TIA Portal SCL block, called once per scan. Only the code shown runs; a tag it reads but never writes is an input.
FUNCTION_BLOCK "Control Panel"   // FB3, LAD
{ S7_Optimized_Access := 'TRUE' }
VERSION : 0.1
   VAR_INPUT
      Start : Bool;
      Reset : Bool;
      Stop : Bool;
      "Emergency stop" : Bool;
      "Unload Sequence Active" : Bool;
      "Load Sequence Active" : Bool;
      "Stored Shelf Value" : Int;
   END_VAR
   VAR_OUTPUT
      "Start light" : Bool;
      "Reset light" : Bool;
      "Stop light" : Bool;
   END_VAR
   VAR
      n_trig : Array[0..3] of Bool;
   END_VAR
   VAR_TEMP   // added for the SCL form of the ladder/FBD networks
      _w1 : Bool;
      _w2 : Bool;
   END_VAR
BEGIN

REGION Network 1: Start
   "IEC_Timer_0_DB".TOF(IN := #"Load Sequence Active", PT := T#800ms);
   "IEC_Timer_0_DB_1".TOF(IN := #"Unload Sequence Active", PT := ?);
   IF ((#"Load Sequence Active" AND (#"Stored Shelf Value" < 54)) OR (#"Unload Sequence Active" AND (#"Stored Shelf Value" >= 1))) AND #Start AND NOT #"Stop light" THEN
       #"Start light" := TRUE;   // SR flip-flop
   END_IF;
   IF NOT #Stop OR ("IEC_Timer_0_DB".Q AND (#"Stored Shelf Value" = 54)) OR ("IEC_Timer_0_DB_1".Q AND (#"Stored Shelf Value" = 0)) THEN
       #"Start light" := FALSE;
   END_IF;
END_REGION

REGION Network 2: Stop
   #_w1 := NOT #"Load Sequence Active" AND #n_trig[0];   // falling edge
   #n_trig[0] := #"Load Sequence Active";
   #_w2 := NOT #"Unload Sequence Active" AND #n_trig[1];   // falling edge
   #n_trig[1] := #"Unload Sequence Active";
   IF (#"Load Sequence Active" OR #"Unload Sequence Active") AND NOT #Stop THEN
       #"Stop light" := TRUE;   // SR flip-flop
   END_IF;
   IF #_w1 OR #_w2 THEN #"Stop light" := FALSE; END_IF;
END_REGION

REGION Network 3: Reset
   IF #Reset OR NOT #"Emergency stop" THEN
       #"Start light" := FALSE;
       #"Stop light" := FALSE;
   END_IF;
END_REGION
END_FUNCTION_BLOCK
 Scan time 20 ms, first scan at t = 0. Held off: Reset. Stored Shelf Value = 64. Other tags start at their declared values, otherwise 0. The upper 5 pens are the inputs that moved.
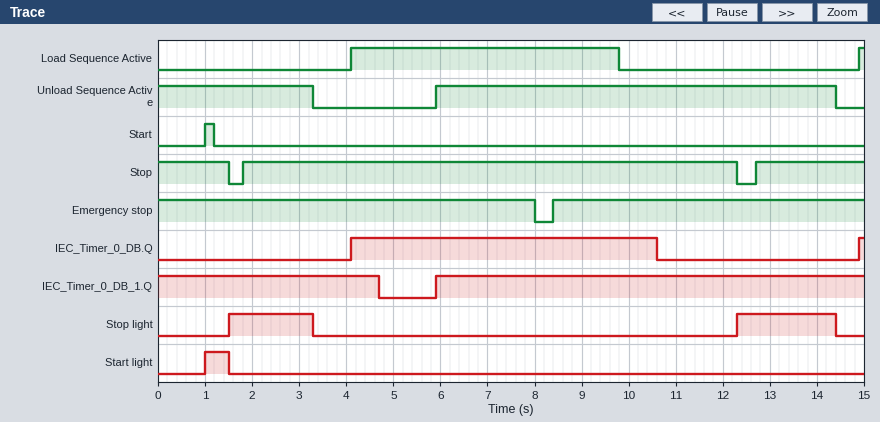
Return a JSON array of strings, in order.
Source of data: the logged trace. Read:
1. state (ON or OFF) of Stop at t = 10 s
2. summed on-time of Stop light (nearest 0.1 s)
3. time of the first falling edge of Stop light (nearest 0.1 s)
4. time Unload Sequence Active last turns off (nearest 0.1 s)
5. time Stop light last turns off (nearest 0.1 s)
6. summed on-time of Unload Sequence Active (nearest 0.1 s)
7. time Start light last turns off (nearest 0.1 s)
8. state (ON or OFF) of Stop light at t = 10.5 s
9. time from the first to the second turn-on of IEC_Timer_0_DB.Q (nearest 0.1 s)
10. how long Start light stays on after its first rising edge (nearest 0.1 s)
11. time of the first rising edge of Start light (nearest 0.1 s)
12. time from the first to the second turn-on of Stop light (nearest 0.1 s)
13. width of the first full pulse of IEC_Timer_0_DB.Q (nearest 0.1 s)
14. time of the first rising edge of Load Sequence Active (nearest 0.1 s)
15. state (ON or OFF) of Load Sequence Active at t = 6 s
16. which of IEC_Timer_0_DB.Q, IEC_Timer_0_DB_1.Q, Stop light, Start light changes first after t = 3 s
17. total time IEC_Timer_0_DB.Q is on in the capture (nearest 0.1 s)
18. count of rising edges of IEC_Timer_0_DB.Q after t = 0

["ON", "3.9 s", "3.3 s", "14.4 s", "14.4 s", "11.8 s", "1.5 s", "OFF", "10.8 s", "0.5 s", "1.0 s", "10.8 s", "6.5 s", "4.1 s", "ON", "Stop light", "6.6 s", "2"]
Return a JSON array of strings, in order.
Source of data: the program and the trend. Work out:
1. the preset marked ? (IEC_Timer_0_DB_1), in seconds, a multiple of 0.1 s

["1.4 s"]
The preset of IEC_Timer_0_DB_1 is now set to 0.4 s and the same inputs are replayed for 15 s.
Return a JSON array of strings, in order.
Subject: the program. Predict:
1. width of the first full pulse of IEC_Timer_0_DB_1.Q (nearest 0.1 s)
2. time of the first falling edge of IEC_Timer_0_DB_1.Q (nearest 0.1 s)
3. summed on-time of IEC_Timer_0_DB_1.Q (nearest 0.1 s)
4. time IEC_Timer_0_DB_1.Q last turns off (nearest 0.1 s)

["8.9 s", "3.7 s", "12.6 s", "14.8 s"]
